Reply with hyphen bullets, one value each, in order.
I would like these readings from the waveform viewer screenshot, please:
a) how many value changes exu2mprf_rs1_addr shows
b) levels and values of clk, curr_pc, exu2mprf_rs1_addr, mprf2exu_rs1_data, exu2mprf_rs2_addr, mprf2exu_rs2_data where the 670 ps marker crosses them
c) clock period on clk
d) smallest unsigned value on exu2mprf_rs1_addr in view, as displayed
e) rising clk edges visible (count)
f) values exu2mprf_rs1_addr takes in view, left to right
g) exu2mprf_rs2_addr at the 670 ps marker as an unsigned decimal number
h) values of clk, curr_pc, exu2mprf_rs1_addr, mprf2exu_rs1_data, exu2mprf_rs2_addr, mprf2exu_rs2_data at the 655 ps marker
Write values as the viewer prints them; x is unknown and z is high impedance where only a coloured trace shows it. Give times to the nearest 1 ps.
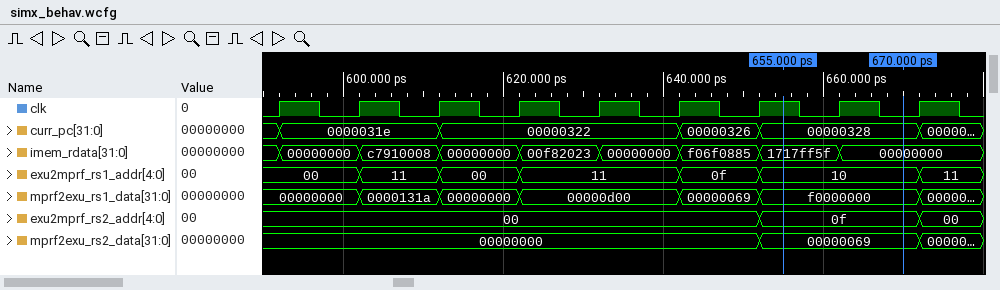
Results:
- 6
- clk=0, curr_pc=00000328, exu2mprf_rs1_addr=10, mprf2exu_rs1_data=f0000000, exu2mprf_rs2_addr=0f, mprf2exu_rs2_data=00000069
- 10 ps
- 00
- 9
- 00, 11, 00, 11, 0f, 10, 11
- 15
- clk=1, curr_pc=00000328, exu2mprf_rs1_addr=10, mprf2exu_rs1_data=f0000000, exu2mprf_rs2_addr=0f, mprf2exu_rs2_data=00000069
